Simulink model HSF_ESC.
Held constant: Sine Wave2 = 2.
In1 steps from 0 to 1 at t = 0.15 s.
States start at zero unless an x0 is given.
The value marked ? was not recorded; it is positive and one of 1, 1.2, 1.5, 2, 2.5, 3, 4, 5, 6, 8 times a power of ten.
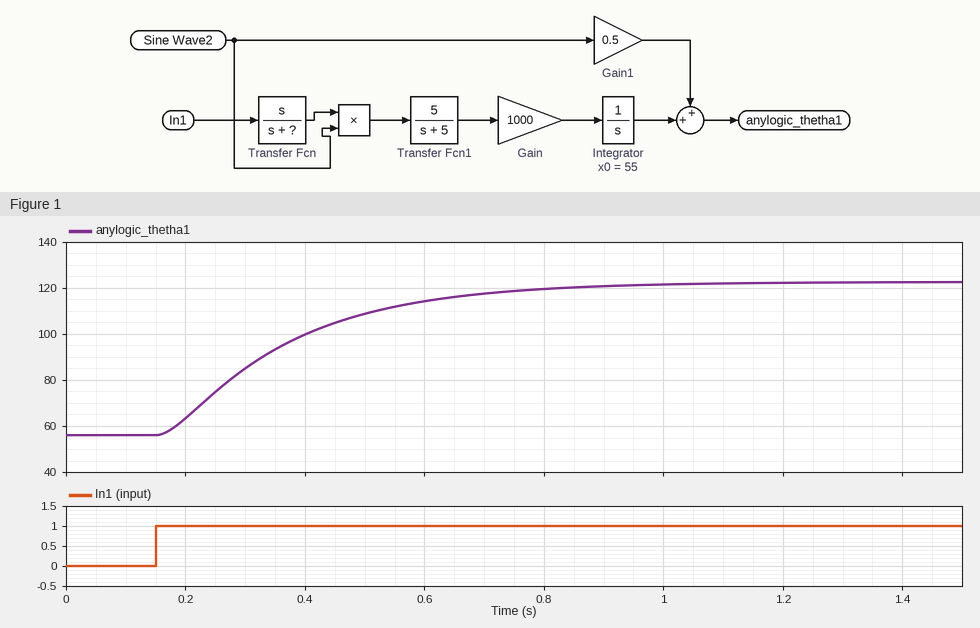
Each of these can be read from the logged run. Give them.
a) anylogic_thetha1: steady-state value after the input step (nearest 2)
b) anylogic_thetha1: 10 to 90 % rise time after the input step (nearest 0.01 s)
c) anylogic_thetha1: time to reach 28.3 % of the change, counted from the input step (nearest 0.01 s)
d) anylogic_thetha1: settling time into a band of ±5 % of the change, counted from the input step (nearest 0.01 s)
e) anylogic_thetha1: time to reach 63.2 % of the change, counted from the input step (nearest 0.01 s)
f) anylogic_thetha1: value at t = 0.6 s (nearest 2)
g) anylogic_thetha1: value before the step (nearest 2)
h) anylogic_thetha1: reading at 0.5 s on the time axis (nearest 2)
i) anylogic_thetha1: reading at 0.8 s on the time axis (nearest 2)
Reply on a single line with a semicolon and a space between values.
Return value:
122; 0.45 s; 0.10 s; 0.64 s; 0.24 s; 114; 56; 108; 120
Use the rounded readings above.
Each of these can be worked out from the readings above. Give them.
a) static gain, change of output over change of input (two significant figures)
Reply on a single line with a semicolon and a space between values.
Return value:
66
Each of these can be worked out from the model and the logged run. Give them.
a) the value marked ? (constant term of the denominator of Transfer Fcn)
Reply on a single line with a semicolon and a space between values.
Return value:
30
